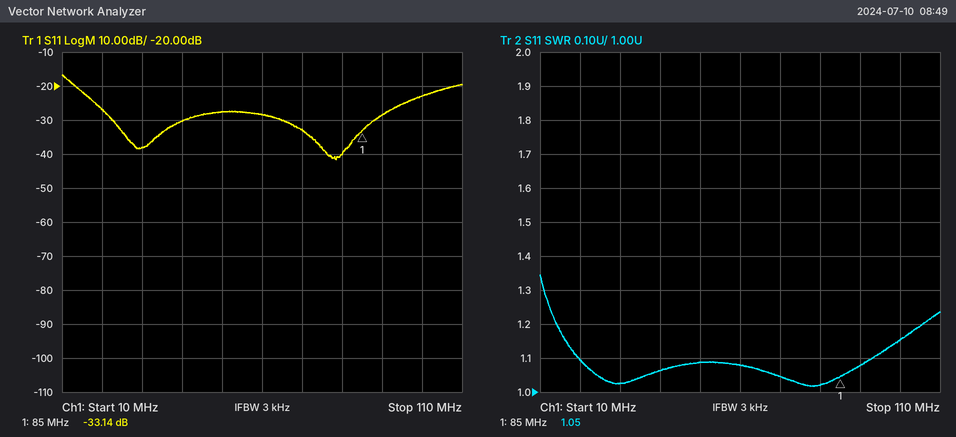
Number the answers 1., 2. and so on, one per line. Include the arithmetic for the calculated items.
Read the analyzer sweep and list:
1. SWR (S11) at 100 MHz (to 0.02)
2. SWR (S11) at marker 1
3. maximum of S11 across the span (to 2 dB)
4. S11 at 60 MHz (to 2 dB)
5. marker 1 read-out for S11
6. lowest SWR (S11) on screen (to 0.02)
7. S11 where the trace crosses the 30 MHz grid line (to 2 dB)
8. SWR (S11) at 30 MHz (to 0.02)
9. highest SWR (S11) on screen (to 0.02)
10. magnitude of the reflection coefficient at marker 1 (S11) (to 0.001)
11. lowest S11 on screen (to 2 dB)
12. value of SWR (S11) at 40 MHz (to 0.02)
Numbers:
1. 1.16
2. 1.05
3. -16 dB
4. -28 dB
5. -33.14 dB
6. 1.02
7. -38 dB
8. 1.02
9. 1.34
10. 10^(-33.14/20) ≈ 0.022
11. -42 dB
12. 1.06
